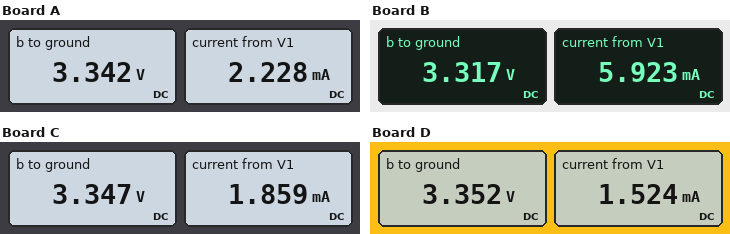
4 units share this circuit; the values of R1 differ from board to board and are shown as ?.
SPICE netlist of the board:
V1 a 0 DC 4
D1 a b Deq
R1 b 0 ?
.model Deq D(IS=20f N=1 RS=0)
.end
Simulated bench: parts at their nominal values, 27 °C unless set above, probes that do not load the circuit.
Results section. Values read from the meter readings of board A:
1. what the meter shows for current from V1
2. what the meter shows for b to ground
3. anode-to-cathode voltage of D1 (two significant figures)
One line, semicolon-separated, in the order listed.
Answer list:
2.228 mA; 3.342 V; 660 mV
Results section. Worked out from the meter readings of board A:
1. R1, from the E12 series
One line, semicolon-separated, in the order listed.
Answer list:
1.5 kΩ
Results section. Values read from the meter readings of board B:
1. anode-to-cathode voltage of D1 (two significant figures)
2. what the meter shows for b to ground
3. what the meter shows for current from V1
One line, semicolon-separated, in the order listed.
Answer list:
680 mV; 3.317 V; 5.923 mA
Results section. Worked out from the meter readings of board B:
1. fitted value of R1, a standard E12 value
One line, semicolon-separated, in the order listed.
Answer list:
560 Ω
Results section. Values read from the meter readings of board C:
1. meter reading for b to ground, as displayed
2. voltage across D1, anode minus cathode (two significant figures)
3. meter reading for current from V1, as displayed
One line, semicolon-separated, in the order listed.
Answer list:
3.347 V; 650 mV; 1.859 mA
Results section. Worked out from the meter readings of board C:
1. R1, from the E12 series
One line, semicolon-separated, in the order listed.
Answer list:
1.8 kΩ
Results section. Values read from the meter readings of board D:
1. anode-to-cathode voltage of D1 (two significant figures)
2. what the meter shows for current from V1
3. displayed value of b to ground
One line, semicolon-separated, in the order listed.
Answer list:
650 mV; 1.524 mA; 3.352 V
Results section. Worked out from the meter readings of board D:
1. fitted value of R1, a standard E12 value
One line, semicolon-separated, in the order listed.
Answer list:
2.2 kΩ
